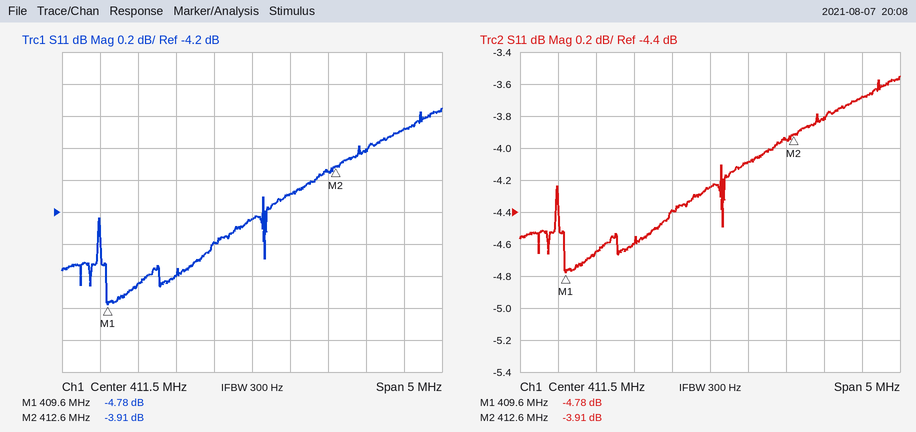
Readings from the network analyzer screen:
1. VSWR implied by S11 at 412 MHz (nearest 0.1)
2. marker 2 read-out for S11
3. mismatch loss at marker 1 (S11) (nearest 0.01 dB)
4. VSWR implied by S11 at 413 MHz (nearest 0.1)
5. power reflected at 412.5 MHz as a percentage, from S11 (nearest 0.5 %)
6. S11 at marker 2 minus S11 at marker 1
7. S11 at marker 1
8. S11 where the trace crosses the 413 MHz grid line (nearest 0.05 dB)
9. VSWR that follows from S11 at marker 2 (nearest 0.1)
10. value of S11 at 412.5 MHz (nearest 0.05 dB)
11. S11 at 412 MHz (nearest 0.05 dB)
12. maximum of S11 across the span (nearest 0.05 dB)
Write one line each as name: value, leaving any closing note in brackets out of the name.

VSWR implied by S11 at 412 MHz: 4.3
marker 2 read-out for S11: -3.91 dB
mismatch loss at marker 1 (S11): 1.76 dB
VSWR implied by S11 at 413 MHz: 4.6
power reflected at 412.5 MHz as a percentage, from S11: 40.5 %
S11 at marker 2 minus S11 at marker 1: 0.87 dB
S11 at marker 1: -4.78 dB
S11 where the trace crosses the 413 MHz grid line: -3.80 dB
VSWR that follows from S11 at marker 2: 4.5
value of S11 at 412.5 MHz: -3.95 dB
S11 at 412 MHz: -4.10 dB
maximum of S11 across the span: -3.55 dB
